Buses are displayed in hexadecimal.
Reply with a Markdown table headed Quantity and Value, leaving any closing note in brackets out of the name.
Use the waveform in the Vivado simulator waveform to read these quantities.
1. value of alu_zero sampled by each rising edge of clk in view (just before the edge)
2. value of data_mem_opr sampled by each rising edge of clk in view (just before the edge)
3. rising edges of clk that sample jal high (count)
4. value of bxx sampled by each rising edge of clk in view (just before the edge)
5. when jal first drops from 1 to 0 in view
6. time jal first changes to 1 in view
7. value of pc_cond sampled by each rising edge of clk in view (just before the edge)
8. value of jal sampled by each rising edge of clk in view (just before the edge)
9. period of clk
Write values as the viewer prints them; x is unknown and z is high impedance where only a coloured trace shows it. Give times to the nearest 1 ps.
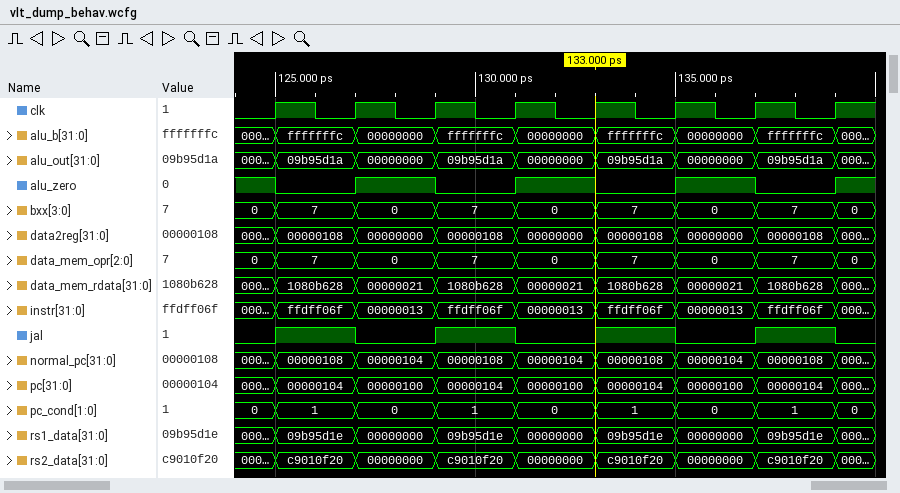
| Quantity | Value |
|---|---|
| value of alu_zero sampled by each rising edge of clk in view | 1 0 1 0 1 0 1 0 |
| value of data_mem_opr sampled by each rising edge of clk in view | 0, 7, 0, 7, 0, 7, 0, 7 |
| rising edges of clk that sample jal high | 4 |
| value of bxx sampled by each rising edge of clk in view | 0, 7, 0, 7, 0, 7, 0, 7 |
| when jal first drops from 1 to 0 in view | 127 ps |
| time jal first changes to 1 in view | 125 ps |
| value of pc_cond sampled by each rising edge of clk in view | 0, 1, 0, 1, 0, 1, 0, 1 |
| value of jal sampled by each rising edge of clk in view | 0 1 0 1 0 1 0 1 |
| period of clk | 2 ps |
